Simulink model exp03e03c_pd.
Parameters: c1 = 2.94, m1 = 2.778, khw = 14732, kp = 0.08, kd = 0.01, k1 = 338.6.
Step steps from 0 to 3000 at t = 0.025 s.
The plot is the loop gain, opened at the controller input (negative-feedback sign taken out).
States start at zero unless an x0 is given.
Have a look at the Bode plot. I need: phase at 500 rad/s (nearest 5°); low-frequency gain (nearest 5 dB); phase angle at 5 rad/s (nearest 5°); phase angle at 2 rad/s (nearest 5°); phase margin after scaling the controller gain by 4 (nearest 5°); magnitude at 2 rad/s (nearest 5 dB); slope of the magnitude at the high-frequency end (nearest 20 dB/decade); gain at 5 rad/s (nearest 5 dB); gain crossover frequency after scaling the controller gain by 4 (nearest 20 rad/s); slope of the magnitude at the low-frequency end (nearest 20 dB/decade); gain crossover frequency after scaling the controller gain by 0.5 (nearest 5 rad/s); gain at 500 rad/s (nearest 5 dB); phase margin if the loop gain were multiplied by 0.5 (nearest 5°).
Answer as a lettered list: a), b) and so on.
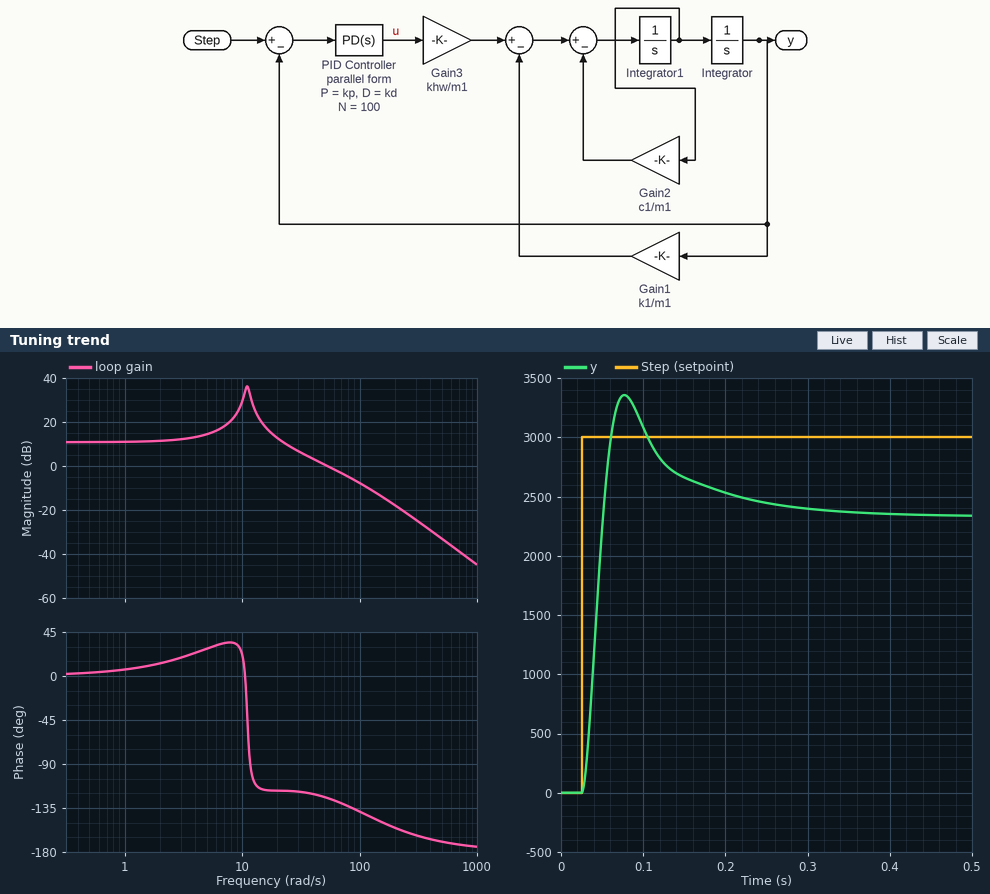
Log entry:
a) -170°
b) 10 dB
c) 30°
d) 15°
e) 35°
f) 10 dB
g) -40 dB/decade
h) 15 dB
i) 140 rad/s
j) 0 dB/decade
k) 30 rad/s
l) -35 dB
m) 60°
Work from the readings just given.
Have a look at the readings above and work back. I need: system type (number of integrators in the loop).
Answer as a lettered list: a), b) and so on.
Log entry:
a) 0
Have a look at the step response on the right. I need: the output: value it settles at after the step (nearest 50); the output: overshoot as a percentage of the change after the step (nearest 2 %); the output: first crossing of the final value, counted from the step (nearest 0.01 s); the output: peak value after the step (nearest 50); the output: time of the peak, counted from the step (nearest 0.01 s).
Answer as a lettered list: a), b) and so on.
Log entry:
a) 2350
b) 44 %
c) 0.03 s
d) 3350
e) 0.05 s
